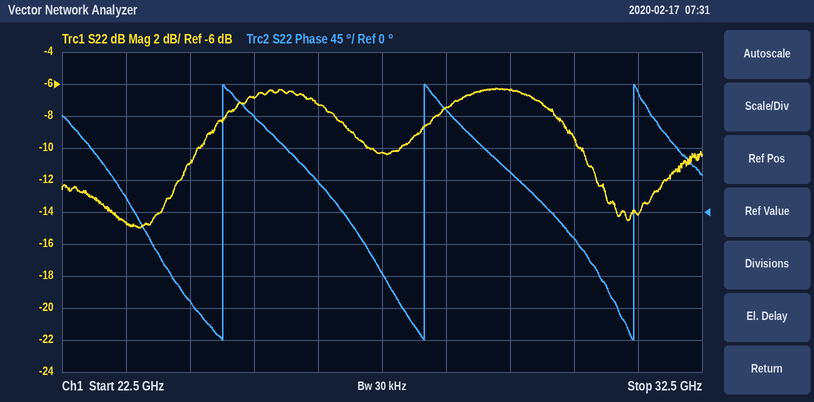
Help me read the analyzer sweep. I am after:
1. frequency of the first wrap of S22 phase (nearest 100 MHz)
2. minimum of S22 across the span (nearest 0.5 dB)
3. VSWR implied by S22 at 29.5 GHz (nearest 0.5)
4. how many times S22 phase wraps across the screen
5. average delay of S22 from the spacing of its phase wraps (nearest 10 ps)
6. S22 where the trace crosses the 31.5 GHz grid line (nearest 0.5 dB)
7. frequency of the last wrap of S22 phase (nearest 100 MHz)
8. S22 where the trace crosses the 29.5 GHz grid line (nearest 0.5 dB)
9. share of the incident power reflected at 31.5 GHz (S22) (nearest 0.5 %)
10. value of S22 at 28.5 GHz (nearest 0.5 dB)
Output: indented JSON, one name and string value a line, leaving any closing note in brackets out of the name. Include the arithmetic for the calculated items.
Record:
{
  "frequency of the first wrap of S22 phase": "25.0 GHz",
  "minimum of S22 across the span": "-15.0 dB",
  "VSWR implied by S22 at 29.5 GHz": "|Γ| = 10^(-6.5/20) = 0.4732; VSWR = (1 + 0.4732)/(1 − 0.4732) ≈ 2.80, so 3.0 to the nearest 0.5",
  "how many times S22 phase wraps across the screen": "3",
  "average delay of S22 from the spacing of its phase wraps": "2 cycles / (31.4 GHz − 25.0 GHz) ≈ 313 ps, so 310 ps to the nearest 10 ps",
  "S22 where the trace crosses the 31.5 GHz grid line": "-14.0 dB",
  "frequency of the last wrap of S22 phase": "31.4 GHz",
  "S22 where the trace crosses the 29.5 GHz grid line": "-6.5 dB",
  "share of the incident power reflected at 31.5 GHz (S22)": "10^(-14/10) ≈ 4.0 %",
  "value of S22 at 28.5 GHz": "-7.5 dB"
}
